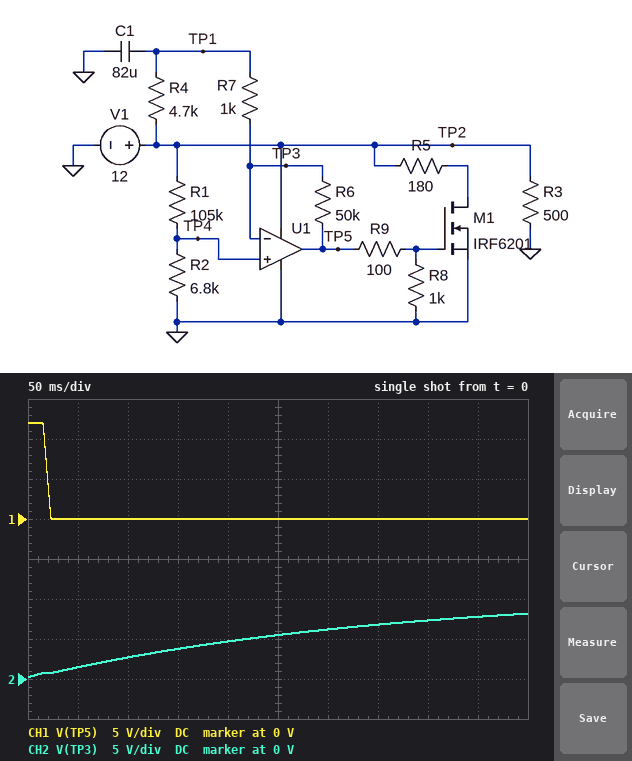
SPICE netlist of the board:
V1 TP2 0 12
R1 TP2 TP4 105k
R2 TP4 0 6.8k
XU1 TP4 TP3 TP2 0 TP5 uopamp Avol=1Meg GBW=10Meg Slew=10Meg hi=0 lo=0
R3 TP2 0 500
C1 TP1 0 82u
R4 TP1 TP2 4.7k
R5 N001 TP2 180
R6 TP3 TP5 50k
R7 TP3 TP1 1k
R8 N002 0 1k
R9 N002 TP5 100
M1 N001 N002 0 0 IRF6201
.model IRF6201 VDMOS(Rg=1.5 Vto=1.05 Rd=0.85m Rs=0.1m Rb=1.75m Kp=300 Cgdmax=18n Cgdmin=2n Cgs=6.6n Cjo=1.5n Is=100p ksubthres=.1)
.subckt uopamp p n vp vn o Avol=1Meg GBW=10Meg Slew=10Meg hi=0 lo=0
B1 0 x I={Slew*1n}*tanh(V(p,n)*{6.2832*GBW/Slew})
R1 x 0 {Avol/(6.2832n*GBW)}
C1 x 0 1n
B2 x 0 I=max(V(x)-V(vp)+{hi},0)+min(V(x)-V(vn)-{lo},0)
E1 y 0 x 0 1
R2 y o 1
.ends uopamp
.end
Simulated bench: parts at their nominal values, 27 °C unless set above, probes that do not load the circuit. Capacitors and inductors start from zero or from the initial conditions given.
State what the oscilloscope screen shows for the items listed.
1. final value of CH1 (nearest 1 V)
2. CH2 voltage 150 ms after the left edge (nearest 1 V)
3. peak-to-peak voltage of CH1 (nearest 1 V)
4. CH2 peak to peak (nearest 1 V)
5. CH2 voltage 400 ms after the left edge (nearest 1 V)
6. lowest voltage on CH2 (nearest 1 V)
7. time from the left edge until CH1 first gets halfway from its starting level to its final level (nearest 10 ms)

0 V
4 V
12 V
8 V
7 V
0 V
20 ms
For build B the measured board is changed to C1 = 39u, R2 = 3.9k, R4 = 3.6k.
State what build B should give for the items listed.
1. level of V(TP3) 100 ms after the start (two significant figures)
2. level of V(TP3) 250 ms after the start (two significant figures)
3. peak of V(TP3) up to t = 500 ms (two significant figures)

5.9 V
9.4 V
11 V
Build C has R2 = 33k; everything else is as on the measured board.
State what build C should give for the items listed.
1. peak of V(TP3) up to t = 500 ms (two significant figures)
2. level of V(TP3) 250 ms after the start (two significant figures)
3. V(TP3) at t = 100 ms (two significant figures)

8.2 V
5.6 V
2.9 V
